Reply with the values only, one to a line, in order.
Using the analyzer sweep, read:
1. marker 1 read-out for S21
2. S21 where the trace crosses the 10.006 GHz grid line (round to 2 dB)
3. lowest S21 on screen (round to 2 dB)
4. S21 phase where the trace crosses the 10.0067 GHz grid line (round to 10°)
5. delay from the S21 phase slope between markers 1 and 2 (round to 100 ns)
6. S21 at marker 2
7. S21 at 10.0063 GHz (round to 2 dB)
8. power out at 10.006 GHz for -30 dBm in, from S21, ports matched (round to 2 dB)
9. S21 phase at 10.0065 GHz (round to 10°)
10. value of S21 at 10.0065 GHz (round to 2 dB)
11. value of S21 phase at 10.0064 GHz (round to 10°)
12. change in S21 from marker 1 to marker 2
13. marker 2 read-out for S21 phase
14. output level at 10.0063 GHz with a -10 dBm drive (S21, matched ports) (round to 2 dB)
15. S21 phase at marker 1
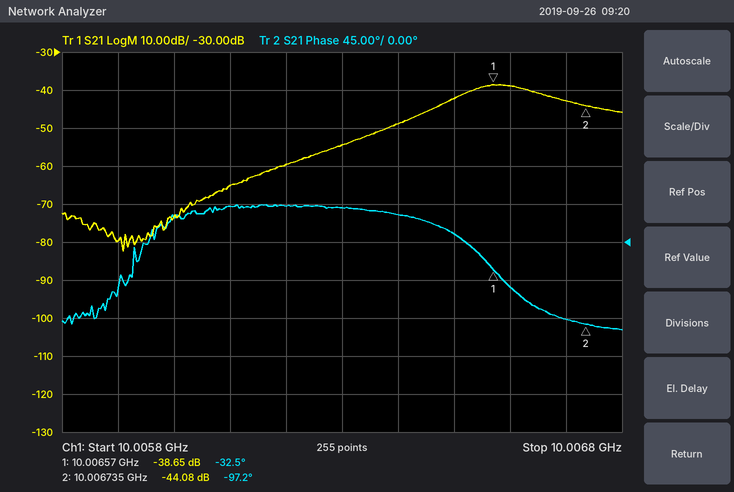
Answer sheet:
-38.65 dB
-74 dB
-82 dB
-90°
1.1 µs
-44.08 dB
-54 dB
-104 dBm
10°
-42 dB
30°
-5.43 dB
-97.2°
-64 dBm
-32.5°
